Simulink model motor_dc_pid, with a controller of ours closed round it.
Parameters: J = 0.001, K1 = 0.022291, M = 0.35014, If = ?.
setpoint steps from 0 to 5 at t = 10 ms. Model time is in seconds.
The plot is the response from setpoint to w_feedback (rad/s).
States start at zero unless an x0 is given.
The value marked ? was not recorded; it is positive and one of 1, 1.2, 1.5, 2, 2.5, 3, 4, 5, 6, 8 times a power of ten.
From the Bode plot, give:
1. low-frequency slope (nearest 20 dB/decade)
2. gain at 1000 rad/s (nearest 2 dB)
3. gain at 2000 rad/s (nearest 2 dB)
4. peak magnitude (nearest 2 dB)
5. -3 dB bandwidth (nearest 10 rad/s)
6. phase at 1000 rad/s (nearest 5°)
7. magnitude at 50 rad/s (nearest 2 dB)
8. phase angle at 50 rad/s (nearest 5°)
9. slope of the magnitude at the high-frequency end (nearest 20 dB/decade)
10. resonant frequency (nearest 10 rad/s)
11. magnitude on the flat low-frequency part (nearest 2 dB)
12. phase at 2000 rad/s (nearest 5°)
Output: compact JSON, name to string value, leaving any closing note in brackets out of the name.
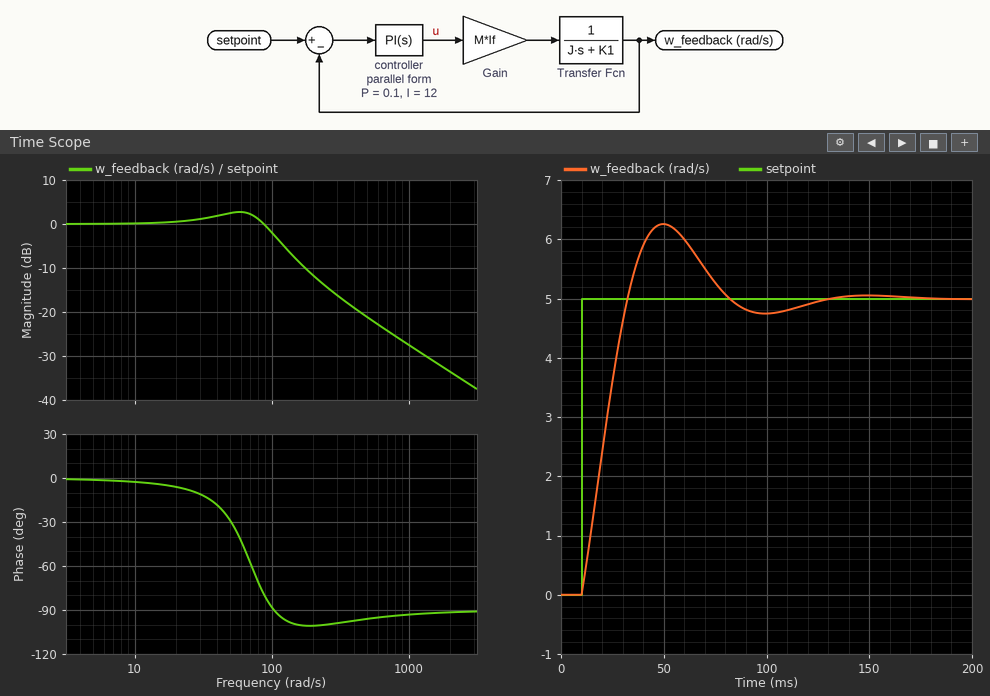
{"low-frequency slope": "0 dB/decade", "gain at 1000 rad/s": "-28 dB", "gain at 2000 rad/s": "-34 dB", "peak magnitude": "2 dB", "-3 dB bandwidth": "110 rad/s", "phase at 1000 rad/s": "-95°", "magnitude at 50 rad/s": "2 dB", "phase angle at 50 rad/s": "-30°", "slope of the magnitude at the high-frequency end": "-20 dB/decade", "resonant frequency": "60 rad/s", "magnitude on the flat low-frequency part": "0 dB", "phase at 2000 rad/s": "-90°"}
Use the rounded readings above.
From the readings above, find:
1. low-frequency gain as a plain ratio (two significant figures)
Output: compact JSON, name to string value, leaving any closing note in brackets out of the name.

{"low-frequency gain as a plain ratio": "1.0"}
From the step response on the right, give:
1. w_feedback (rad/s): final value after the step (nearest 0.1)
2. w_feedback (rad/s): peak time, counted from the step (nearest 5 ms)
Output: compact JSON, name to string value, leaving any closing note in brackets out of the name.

{"w_feedback (rad/s): final value after the step": "5.0", "w_feedback (rad/s): peak time, counted from the step": "40 ms"}
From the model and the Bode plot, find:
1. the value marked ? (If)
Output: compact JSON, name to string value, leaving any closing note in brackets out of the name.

{"the value marked ?": "1.2"}
